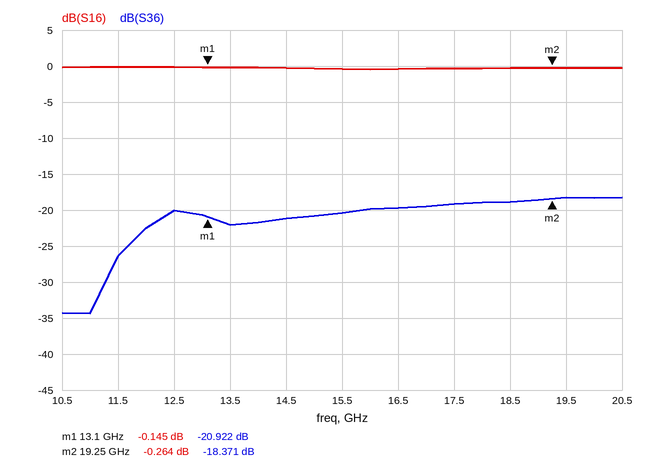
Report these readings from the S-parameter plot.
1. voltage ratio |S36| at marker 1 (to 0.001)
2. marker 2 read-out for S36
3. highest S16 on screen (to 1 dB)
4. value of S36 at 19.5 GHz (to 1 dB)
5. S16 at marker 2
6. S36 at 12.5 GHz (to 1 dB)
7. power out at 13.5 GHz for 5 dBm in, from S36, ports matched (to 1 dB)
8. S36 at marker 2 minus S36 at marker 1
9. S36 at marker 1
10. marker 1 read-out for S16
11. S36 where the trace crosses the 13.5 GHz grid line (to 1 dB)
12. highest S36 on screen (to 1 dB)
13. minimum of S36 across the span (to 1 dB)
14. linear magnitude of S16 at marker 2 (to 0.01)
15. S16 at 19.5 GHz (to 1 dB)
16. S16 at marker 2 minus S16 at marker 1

0.090
-18.371 dB
0 dB
-18 dB
-0.264 dB
-20 dB
-17 dBm
2.551 dB
-20.922 dB
-0.145 dB
-22 dB
-18 dB
-34 dB
0.97
0 dB
-0.119 dB
